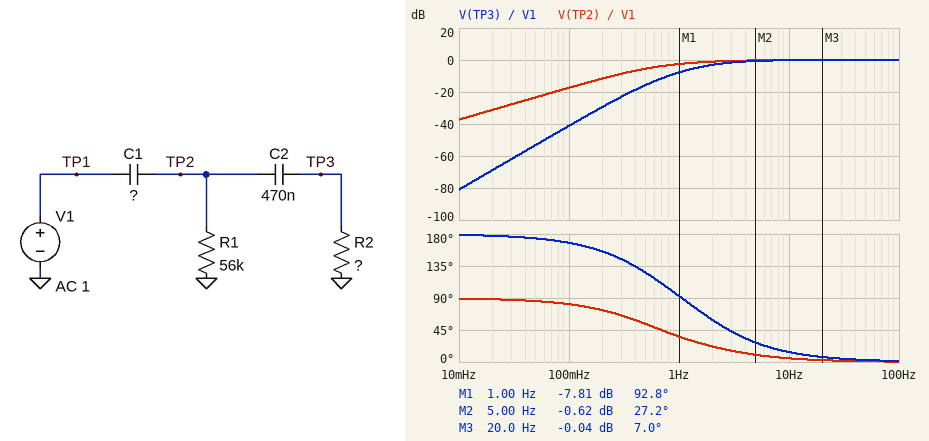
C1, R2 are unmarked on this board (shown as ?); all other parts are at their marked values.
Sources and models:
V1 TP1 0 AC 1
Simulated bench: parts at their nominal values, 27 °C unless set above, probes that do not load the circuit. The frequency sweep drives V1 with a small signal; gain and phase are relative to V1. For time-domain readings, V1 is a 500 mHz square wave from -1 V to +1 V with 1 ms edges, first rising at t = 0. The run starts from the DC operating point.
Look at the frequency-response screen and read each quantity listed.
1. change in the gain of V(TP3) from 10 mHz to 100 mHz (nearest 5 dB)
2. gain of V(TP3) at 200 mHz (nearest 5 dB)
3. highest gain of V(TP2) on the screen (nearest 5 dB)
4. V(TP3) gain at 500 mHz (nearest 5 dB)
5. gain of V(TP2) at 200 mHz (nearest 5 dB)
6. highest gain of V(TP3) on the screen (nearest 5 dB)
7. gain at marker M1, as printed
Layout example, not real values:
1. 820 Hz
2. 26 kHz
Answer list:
1. 40 dB
2. -30 dB
3. 0 dB
4. -15 dB
5. -10 dB
6. 0 dB
7. -7.81 dB
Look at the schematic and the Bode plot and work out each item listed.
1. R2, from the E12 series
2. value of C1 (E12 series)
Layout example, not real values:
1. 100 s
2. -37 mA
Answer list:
1. 220 kΩ
2. 3.9 µF
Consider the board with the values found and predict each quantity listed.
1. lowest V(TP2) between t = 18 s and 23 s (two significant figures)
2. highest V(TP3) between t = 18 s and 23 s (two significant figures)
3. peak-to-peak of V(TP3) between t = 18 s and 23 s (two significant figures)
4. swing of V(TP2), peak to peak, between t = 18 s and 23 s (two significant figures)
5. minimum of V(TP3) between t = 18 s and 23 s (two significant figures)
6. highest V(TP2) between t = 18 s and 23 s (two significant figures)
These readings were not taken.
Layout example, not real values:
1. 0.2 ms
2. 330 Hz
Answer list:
1. -2.0 V
2. 2.0 V
3. 4.0 V
4. 3.9 V
5. -2.0 V
6. 2.0 V
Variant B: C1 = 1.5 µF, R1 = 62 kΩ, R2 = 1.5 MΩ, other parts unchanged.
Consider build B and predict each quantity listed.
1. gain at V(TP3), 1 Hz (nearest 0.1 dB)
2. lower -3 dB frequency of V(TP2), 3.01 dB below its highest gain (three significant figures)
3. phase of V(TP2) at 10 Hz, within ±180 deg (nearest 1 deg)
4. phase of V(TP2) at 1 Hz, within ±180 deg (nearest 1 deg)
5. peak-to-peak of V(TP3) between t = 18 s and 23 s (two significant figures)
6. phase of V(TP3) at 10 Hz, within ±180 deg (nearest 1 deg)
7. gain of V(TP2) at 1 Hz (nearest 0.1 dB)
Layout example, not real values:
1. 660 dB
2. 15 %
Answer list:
1. -6.4 dB
2. 1.79 Hz
3. 10 deg
4. 60 deg
5. 4.1 V
6. 11 deg
7. -6.2 dB
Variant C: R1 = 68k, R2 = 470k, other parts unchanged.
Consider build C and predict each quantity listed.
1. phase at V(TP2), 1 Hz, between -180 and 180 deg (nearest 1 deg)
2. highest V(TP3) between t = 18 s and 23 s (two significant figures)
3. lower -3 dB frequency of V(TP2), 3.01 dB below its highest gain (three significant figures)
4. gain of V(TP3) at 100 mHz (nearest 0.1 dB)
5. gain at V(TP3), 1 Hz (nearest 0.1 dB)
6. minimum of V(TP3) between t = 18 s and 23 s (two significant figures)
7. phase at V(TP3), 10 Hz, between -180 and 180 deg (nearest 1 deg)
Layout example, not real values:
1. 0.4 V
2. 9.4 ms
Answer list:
1. 32 deg
2. 2.1 V
3. 688 mHz
4. -33.0 dB
5. -3.6 dB
6. -2.1 V
7. 8 deg
